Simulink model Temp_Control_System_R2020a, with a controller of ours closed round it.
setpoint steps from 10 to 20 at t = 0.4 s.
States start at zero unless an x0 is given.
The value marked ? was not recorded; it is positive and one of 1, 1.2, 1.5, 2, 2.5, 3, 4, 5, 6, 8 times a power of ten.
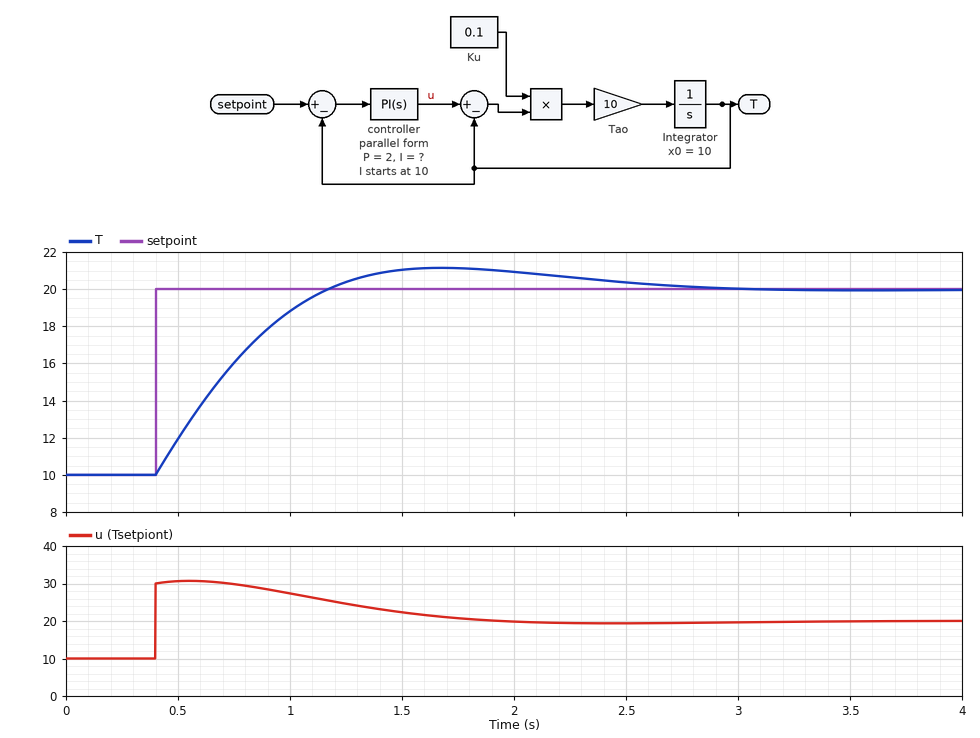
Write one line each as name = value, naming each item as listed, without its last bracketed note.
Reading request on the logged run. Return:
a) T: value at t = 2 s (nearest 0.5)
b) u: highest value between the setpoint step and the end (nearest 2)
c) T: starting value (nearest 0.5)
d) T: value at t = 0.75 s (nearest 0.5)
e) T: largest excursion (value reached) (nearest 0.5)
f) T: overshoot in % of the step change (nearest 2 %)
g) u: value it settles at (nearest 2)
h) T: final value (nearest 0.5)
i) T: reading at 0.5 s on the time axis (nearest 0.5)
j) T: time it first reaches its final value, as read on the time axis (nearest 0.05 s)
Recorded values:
T: value at t = 2 s = 21.0
u: highest value between the setpoint step and the end = 30
T: starting value = 10.0
T: value at t = 0.75 s = 16.0
T: largest excursion (value reached) = 21.0
T: overshoot in % of the step change = 12 %
u: value it settles at = 20
T: final value = 20.0
T: reading at 0.5 s on the time axis = 12.0
T: time it first reaches its final value, as read on the time axis = 1.15 s
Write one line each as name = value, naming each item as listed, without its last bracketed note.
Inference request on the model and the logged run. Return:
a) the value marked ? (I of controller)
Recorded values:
the value marked ? = 5
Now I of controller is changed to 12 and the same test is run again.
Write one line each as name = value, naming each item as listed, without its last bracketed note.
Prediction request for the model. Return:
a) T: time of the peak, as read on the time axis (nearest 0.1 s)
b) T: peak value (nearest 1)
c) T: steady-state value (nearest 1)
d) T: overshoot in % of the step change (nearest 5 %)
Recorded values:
T: time of the peak, as read on the time axis = 1.2 s
T: peak value = 23
T: steady-state value = 20
T: overshoot in % of the step change = 25 %
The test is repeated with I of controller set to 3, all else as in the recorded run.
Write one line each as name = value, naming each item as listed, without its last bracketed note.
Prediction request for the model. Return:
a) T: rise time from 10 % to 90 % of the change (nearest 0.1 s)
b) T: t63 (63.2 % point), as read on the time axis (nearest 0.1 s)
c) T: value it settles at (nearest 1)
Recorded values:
T: rise time from 10 % to 90 % of the change = 0.8 s
T: t63 (63.2 % point), as read on the time axis = 0.8 s
T: value it settles at = 20
